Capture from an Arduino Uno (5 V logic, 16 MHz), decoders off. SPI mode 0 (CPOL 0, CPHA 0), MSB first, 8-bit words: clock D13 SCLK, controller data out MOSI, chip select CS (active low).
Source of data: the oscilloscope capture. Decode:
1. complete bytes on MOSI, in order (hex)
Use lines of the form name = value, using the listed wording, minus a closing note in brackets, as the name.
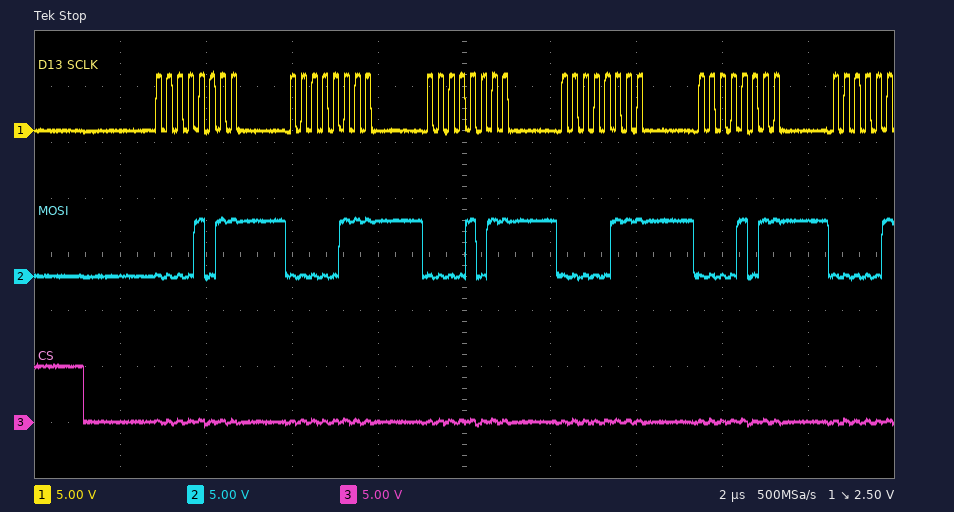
complete bytes on MOSI, in order = 0x0B 0x07 0x0B 0x07 0x0B
